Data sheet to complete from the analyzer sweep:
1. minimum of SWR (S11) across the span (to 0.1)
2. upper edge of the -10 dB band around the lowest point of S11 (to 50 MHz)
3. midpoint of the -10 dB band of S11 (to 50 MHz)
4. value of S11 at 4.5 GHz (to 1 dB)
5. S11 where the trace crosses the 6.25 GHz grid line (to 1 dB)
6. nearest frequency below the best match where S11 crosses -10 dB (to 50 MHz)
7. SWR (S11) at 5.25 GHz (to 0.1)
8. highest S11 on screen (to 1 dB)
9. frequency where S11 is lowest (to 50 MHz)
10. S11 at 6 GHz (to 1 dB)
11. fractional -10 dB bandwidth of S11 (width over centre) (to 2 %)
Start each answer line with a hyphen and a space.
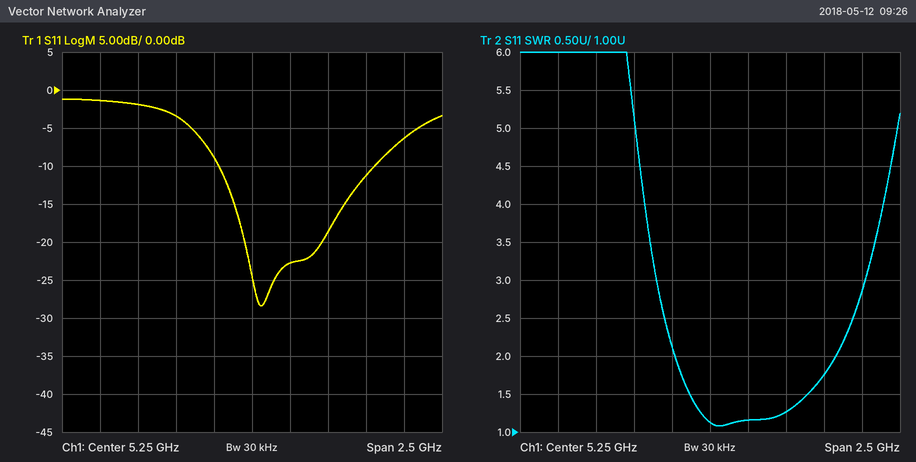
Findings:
- 1.1
- 6.05 GHz
- 5.55 GHz
- -2 dB
- -6 dB
- 5.05 GHz
- 1.1
- -1 dB
- 5.30 GHz
- -11 dB
- 18 %
